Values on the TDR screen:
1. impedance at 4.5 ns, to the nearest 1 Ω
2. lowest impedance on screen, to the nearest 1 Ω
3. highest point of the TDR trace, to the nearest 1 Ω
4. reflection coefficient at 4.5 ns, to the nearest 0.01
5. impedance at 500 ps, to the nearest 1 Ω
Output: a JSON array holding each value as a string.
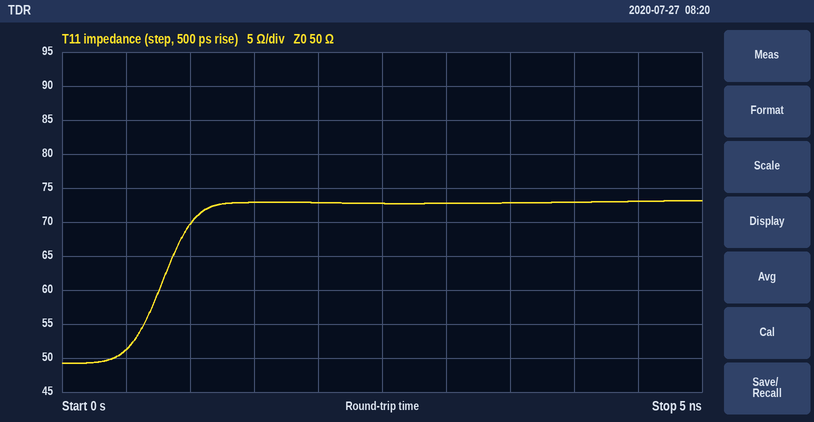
["73 Ω", "49 Ω", "73 Ω", "+0.19", "51 Ω"]
